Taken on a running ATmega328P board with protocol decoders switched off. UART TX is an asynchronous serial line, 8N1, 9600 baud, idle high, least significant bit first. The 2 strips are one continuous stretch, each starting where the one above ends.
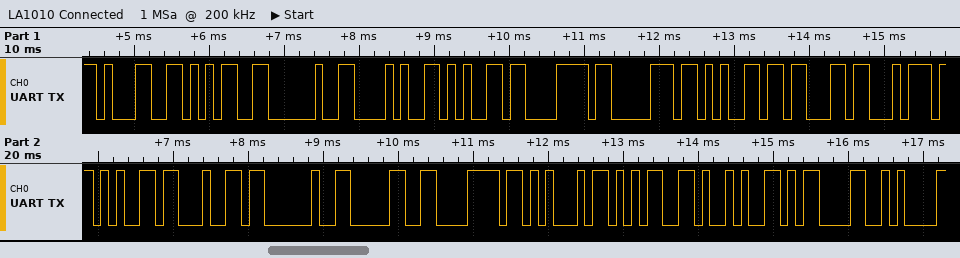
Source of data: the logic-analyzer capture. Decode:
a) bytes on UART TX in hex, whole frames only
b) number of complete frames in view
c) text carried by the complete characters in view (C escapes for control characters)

0x31 0x35 0x20 0x28 0x65 0x78 0x70 0x65 0x63 0x74 0x65 0x64 0x20 0x30 0x78 0x45 0x35 0x29 0x0D 0x0A
20
"15 (expected 0xE5)\r\n"
